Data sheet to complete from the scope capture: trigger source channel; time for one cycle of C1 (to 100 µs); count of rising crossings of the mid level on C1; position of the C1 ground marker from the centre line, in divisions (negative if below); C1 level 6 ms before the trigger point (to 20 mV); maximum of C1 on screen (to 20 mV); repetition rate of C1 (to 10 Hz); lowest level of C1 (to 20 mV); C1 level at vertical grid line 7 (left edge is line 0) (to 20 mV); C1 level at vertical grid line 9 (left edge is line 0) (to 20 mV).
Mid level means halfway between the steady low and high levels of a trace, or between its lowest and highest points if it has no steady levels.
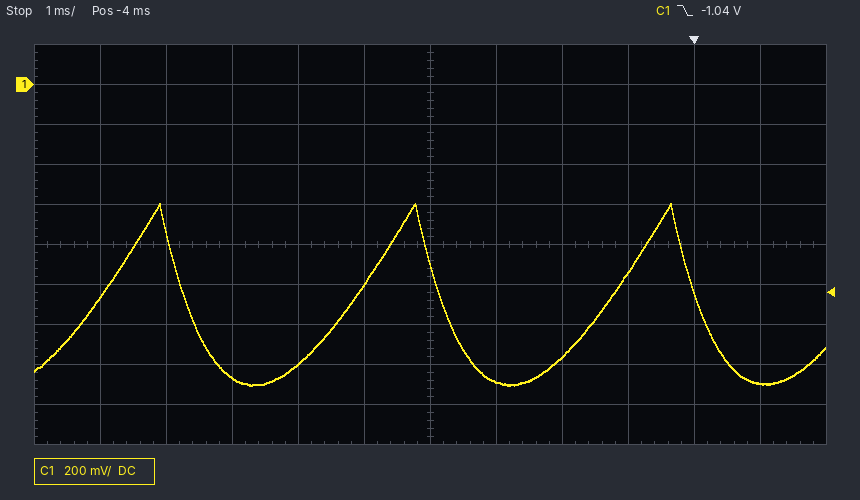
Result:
C1
3.9 ms
3
+4.0 div
-1.40 V
-600 mV
260 Hz
-1.50 V
-1.48 V
-940 mV
